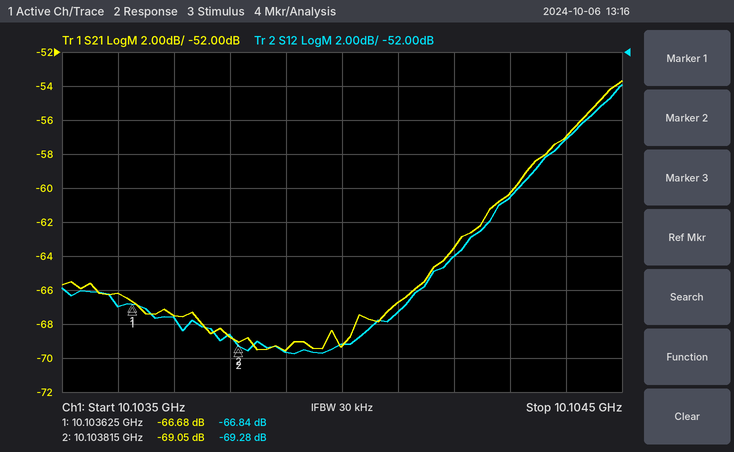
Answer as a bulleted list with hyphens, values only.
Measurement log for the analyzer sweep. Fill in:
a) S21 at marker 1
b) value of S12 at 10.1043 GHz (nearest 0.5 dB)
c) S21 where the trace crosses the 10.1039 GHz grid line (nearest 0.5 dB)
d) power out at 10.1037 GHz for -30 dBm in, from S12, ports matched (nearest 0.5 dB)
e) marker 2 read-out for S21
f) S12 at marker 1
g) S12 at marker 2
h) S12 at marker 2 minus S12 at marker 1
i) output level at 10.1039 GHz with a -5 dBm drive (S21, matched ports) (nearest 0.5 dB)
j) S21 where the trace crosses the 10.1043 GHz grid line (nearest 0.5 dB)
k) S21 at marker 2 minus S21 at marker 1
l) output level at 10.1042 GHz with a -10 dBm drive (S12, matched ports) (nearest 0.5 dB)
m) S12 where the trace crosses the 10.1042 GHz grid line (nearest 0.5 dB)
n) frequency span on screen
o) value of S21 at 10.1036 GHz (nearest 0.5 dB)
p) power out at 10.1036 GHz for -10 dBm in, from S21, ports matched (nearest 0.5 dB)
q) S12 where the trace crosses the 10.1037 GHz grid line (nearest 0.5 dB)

- -66.68 dB
- -60.5 dB
- -69.5 dB
- -97.5 dBm
- -69.05 dB
- -66.84 dB
- -69.28 dB
- -2.44 dB
- -74.5 dBm
- -60.5 dB
- -2.37 dB
- -74.0 dBm
- -64.0 dB
- 1 MHz
- -66.0 dB
- -76.0 dBm
- -67.5 dB
